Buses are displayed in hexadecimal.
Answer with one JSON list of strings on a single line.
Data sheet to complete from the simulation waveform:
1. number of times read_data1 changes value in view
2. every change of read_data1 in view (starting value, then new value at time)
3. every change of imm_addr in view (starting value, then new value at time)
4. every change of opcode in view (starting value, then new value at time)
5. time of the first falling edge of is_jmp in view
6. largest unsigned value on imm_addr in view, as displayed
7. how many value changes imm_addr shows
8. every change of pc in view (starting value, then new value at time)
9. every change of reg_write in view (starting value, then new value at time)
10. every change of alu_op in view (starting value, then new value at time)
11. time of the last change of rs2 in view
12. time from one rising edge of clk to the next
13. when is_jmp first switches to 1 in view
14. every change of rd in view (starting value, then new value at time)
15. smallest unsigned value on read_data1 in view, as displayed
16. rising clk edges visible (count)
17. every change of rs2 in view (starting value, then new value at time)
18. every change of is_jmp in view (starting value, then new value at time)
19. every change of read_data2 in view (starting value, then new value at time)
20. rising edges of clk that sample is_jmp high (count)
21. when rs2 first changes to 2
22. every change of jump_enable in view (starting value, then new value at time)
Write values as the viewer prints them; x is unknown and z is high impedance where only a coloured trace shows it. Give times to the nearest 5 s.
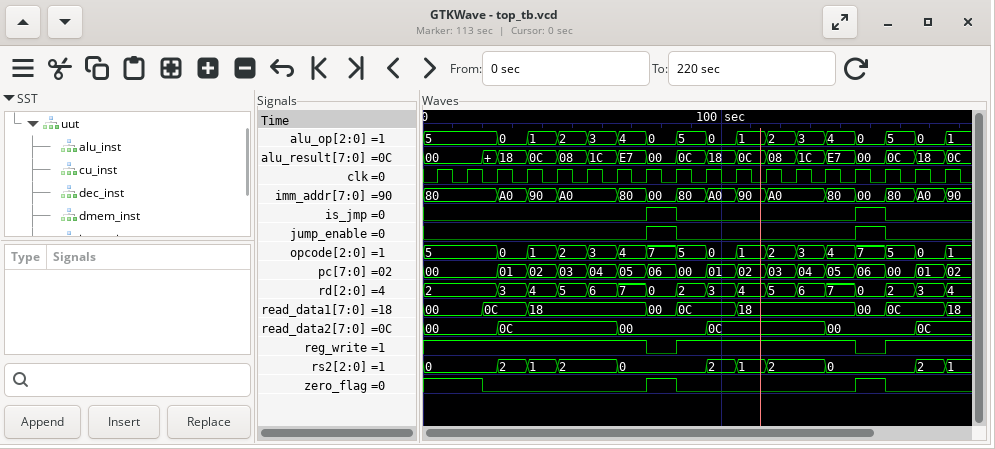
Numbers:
["8", "00, 0C at 20 s, 18 at 35 s, 00 at 75 s, 0C at 85 s, 18 at 105 s, 00 at 145 s, 0C at 155 s, 18 at 175 s", "80, A0 at 25 s, 90 at 35 s, A0 at 45 s, 80 at 65 s, 00 at 75 s, 80 at 85 s, A0 at 95 s, 90 at 105 s, A0 at 115 s, 80 at 135 s, 00 at 145 s, 80 at 155 s, A0 at 165 s, 90 at 175 s", "5, 0 at 25 s, 1 at 35 s, 2 at 45 s, 3 at 55 s, 4 at 65 s, 7 at 75 s, 5 at 85 s, 0 at 95 s, 1 at 105 s, 2 at 115 s, 3 at 125 s, 4 at 135 s, 7 at 145 s, 5 at 155 s, 0 at 165 s, 1 at 175 s", "85 s", "A0", "14", "00, 01 at 25 s, 02 at 35 s, 03 at 45 s, 04 at 55 s, 05 at 65 s, 06 at 75 s, 00 at 85 s, 01 at 95 s, 02 at 105 s, 03 at 115 s, 04 at 125 s, 05 at 135 s, 06 at 145 s, 00 at 155 s, 01 at 165 s, 02 at 175 s", "1, 0 at 75 s, 1 at 85 s, 0 at 145 s, 1 at 155 s", "5, 0 at 25 s, 1 at 35 s, 2 at 45 s, 3 at 55 s, 4 at 65 s, 0 at 75 s, 5 at 85 s, 0 at 95 s, 1 at 105 s, 2 at 115 s, 3 at 125 s, 4 at 135 s, 0 at 145 s, 5 at 155 s, 0 at 165 s, 1 at 175 s", "175 s", "10 s", "75 s", "2, 3 at 25 s, 4 at 35 s, 5 at 45 s, 6 at 55 s, 7 at 65 s, 0 at 75 s, 2 at 85 s, 3 at 95 s, 4 at 105 s, 5 at 115 s, 6 at 125 s, 7 at 135 s, 0 at 145 s, 2 at 155 s, 3 at 165 s, 4 at 175 s", "00", "18", "0, 2 at 25 s, 1 at 35 s, 2 at 45 s, 0 at 65 s, 2 at 95 s, 1 at 105 s, 2 at 115 s, 0 at 135 s, 2 at 165 s, 1 at 175 s", "0, 1 at 75 s, 0 at 85 s, 1 at 145 s, 0 at 155 s", "00, 0C at 25 s, 00 at 65 s, 0C at 95 s, 00 at 135 s, 0C at 165 s", "2", "25 s", "0, 1 at 75 s, 0 at 85 s, 1 at 145 s, 0 at 155 s"]
